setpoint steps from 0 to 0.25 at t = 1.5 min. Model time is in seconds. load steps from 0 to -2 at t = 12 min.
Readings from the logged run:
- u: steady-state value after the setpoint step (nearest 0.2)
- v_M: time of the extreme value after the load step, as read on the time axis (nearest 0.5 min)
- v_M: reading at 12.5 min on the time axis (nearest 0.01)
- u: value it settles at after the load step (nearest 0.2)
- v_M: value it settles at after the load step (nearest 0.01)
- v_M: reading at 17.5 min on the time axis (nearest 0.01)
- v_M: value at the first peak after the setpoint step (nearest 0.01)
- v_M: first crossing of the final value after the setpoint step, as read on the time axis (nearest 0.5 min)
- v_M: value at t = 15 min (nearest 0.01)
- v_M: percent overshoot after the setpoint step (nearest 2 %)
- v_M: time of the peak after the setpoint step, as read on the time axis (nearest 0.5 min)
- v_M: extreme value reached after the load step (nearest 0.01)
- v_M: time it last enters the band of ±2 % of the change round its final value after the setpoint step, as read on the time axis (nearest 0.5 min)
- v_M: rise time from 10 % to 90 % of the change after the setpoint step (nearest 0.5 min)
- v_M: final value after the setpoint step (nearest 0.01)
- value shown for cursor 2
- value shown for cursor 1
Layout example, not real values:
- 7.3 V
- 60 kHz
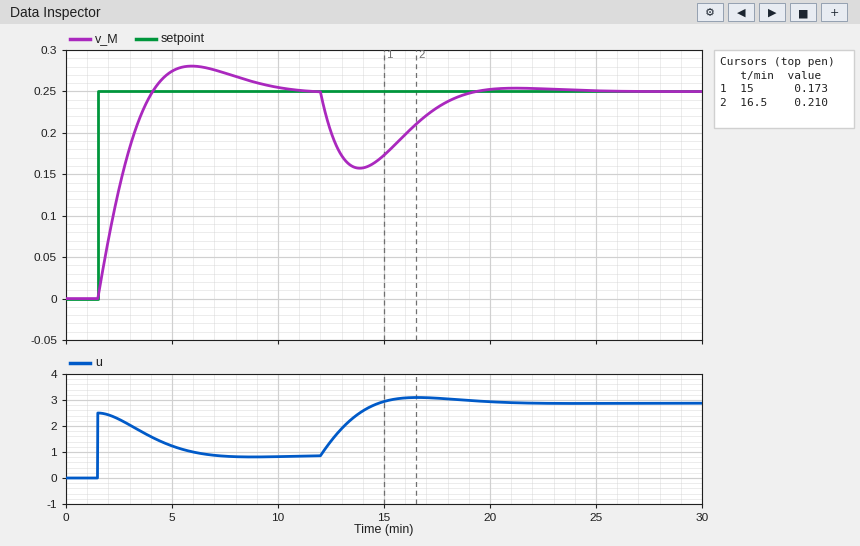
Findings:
- 0.8
- 14.0 min
- 0.20
- 2.8
- 0.25
- 0.23
- 0.28
- 4.0 min
- 0.17
- 12 %
- 6.0 min
- 0.16
- 10.0 min
- 2.0 min
- 0.25
- 0.210
- 0.173
